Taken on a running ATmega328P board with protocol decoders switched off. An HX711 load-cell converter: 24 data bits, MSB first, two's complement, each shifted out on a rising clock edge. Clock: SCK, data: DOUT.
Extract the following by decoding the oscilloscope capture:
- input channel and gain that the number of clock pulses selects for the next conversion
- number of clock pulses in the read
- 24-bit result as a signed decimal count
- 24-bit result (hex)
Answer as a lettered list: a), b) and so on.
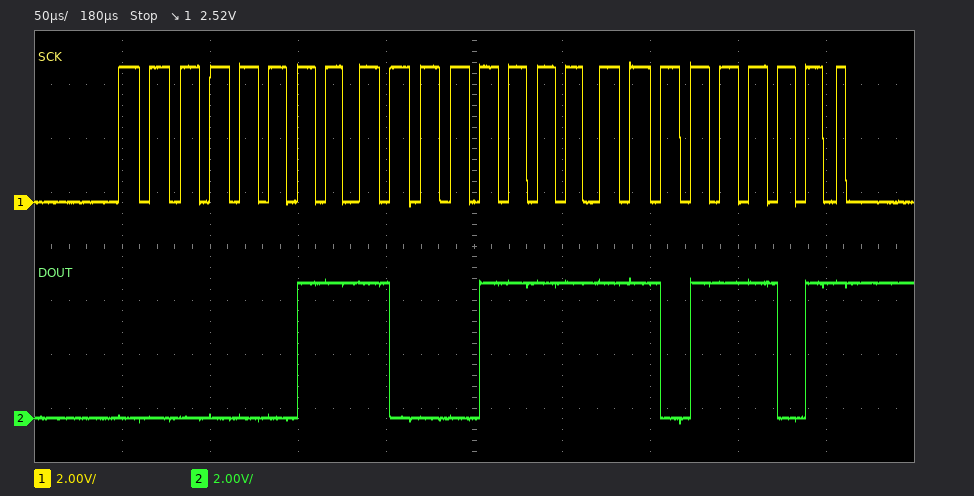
a) channel A, gain 128
b) 25
c) 233437
d) 0x038FDD
